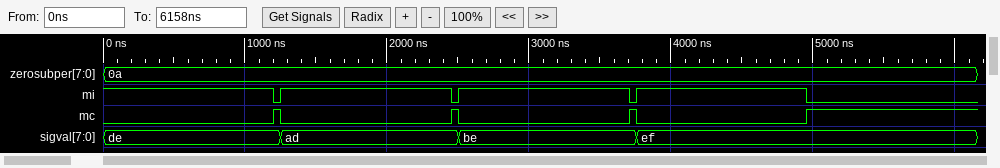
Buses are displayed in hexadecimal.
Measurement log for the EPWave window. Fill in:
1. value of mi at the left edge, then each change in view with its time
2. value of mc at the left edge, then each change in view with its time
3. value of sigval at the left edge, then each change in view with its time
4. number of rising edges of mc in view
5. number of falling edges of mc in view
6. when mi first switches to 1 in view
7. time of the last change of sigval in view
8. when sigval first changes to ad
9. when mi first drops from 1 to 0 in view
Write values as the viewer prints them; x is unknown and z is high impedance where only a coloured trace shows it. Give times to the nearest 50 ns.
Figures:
1, 0 at 1200 ns, 1 at 1250 ns, 0 at 2450 ns, 1 at 2500 ns, 0 at 3700 ns, 1 at 3750 ns, 0 at 4950 ns
0, 1 at 1200 ns, 0 at 1250 ns, 1 at 2450 ns, 0 at 2500 ns, 1 at 3700 ns, 0 at 3750 ns, 1 at 4950 ns
de, ad at 1250 ns, be at 2500 ns, ef at 3750 ns
4
3
1250 ns
3750 ns
1250 ns
1200 ns
